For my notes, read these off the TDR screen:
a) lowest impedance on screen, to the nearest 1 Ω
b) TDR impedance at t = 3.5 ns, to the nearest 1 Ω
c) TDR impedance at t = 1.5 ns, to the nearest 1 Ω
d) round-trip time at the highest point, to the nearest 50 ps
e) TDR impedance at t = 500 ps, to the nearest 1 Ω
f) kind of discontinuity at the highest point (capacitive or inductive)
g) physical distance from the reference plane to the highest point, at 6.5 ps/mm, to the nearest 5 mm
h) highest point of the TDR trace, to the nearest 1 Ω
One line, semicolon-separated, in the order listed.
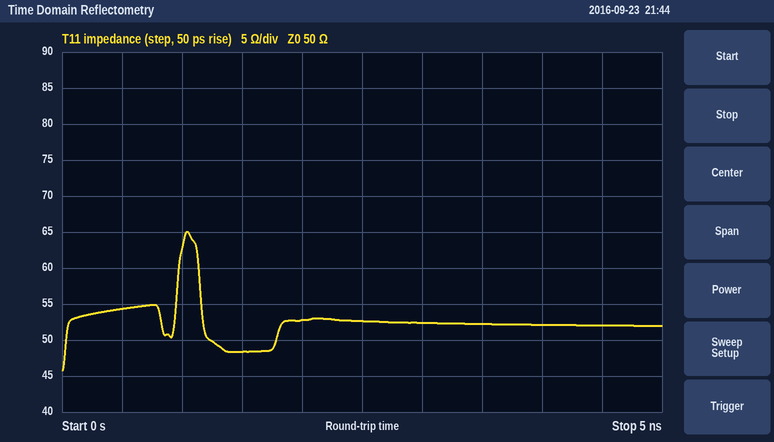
46 Ω; 52 Ω; 48 Ω; 1.05 ns; 54 Ω; inductive; 80 mm; 65 Ω
